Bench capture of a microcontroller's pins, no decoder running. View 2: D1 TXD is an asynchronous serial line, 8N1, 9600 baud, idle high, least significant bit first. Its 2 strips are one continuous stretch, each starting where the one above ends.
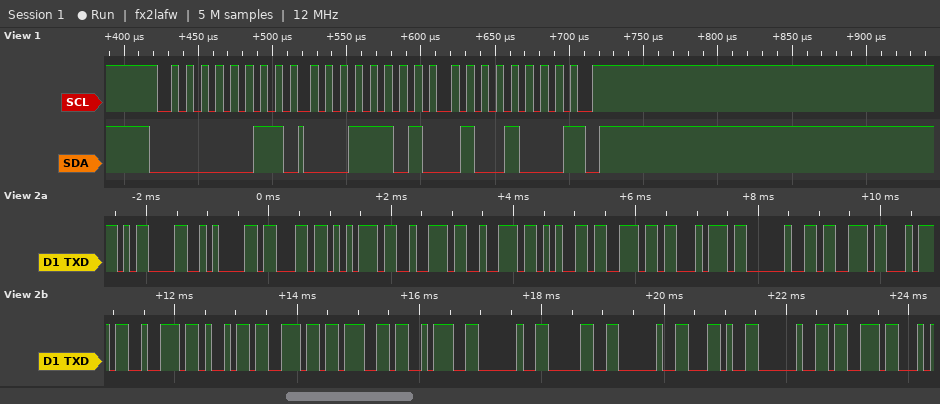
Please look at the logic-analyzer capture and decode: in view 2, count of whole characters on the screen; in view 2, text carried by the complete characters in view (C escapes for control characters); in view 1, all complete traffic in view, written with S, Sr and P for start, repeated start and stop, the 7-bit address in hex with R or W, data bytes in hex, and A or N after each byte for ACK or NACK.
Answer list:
23
"\r\ncurrent string: 0 , s"
S 01R A 1D A 48 N P
